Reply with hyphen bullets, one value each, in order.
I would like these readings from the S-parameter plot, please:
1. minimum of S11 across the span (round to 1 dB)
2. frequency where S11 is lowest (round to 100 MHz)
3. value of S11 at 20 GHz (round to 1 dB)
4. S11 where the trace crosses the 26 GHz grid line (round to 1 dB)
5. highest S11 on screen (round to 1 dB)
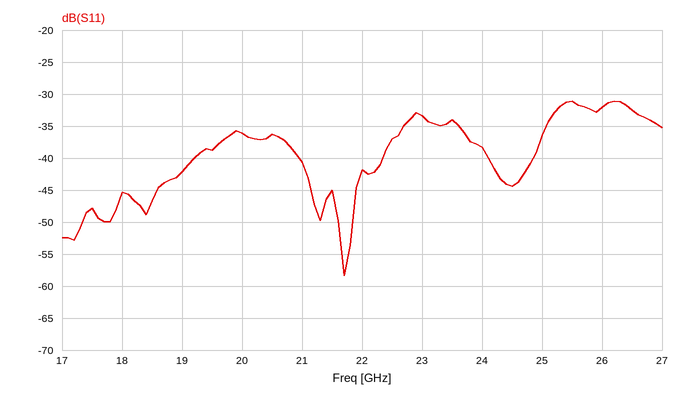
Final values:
- -58 dB
- 21.7 GHz
- -36 dB
- -32 dB
- -31 dB
